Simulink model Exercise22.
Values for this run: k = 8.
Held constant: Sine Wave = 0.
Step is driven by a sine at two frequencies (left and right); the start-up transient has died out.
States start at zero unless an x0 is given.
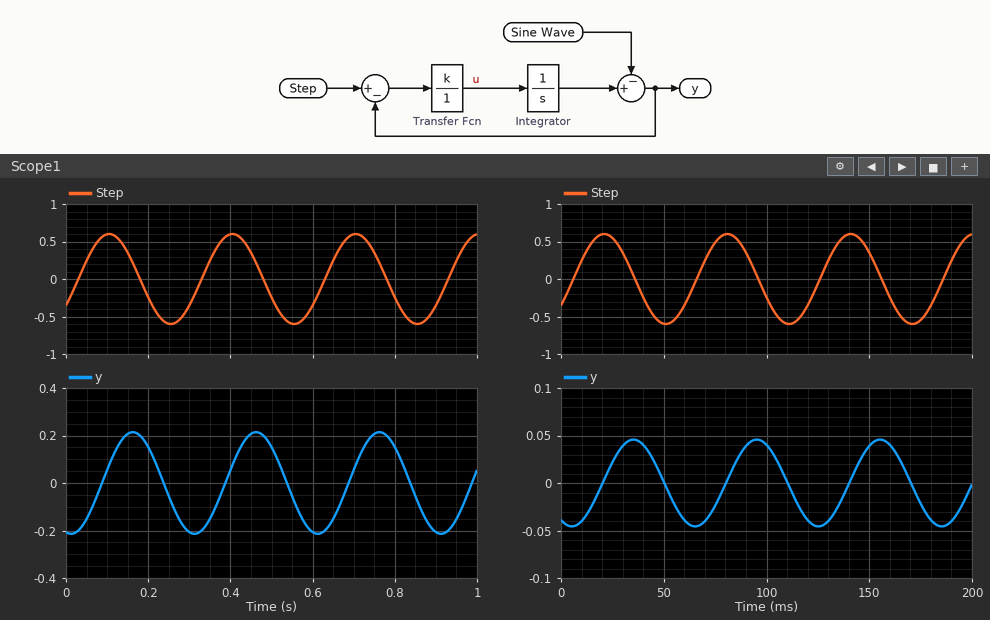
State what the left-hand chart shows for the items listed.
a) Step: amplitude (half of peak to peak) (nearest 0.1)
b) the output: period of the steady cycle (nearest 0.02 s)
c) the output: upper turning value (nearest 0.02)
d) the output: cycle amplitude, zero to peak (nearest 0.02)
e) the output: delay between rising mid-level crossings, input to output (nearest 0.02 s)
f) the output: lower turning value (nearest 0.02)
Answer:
0.6
0.30 s
0.22
0.22
0.06 s
-0.22
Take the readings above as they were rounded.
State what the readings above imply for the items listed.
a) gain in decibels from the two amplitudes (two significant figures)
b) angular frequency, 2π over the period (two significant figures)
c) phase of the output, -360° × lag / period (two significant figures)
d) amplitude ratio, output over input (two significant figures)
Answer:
-8.7 dB
21 rad/s
-72°
0.37
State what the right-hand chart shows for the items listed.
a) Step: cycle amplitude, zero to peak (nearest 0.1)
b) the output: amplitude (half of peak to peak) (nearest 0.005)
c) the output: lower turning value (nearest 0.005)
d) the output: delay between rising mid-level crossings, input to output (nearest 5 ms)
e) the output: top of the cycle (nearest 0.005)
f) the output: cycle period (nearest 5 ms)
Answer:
0.6
0.045
-0.045
15 ms
0.045
60 ms
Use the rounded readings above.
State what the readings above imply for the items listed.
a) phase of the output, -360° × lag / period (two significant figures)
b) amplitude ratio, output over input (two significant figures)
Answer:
-90°
0.075
